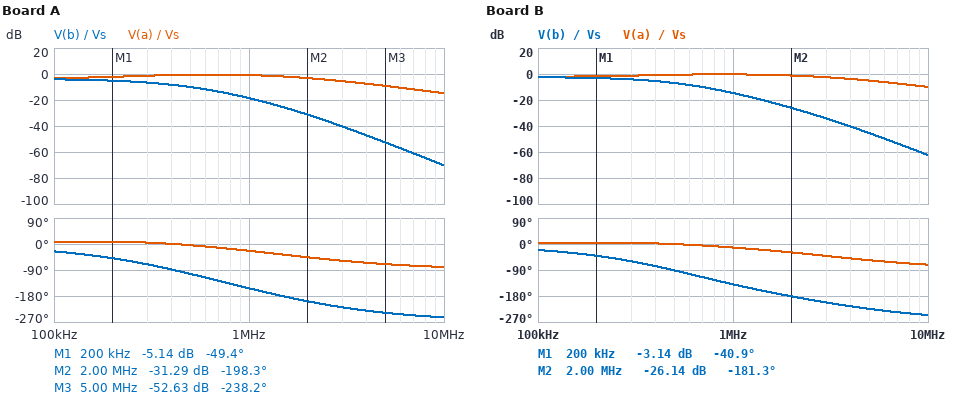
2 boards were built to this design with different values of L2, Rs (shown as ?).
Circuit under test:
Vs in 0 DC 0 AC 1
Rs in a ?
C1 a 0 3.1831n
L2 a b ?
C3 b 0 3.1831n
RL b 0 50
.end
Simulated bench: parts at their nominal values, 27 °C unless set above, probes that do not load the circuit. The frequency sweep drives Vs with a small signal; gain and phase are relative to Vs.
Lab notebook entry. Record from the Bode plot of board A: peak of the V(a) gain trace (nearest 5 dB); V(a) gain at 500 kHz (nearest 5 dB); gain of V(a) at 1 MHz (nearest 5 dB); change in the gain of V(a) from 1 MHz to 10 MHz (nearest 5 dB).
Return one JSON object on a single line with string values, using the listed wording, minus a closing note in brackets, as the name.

{"peak of the V(a) gain trace": "0 dB", "V(a) gain at 500 kHz": "0 dB", "gain of V(a) at 1 MHz": "0 dB", "change in the gain of V(a) from 1 MHz to 10 MHz": "-15 dB"}
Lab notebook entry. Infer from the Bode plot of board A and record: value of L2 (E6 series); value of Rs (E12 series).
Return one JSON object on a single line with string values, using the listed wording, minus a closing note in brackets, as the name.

{"value of L2": "47 µH", "value of Rs": "27 Ω"}
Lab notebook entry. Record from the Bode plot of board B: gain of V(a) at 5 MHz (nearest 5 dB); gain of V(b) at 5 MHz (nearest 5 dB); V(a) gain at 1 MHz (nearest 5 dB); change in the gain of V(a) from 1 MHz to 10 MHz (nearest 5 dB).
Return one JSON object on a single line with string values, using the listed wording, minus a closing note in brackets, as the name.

{"gain of V(a) at 5 MHz": "-5 dB", "gain of V(b) at 5 MHz": "-45 dB", "V(a) gain at 1 MHz": "0 dB", "change in the gain of V(a) from 1 MHz to 10 MHz": "-10 dB"}
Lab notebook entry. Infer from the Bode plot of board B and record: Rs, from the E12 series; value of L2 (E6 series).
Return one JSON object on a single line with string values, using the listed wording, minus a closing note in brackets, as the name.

{"Rs, from the E12 series": "15 Ω", "value of L2": "33 µH"}
